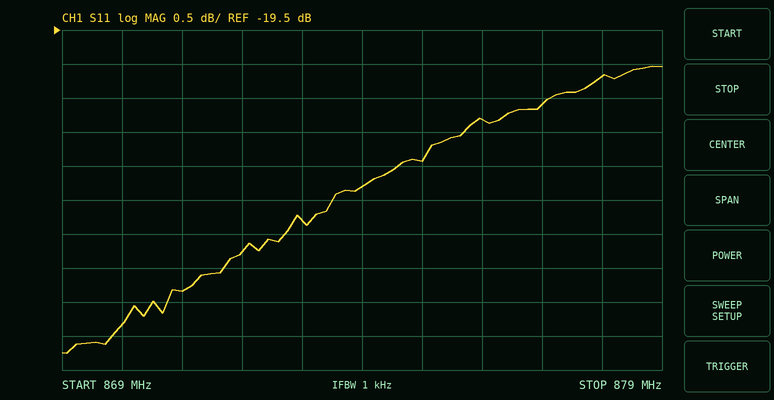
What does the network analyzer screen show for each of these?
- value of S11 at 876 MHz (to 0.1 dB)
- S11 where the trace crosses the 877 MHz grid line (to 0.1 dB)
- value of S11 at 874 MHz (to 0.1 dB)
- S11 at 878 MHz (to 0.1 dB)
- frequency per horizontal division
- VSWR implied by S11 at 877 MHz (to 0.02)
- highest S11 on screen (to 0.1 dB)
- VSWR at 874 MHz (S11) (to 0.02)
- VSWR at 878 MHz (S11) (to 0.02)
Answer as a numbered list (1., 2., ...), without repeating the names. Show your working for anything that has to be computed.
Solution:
1. -20.8 dB
2. -20.6 dB
3. -21.8 dB
4. -20.2 dB
5. 1 MHz
6. |Γ| = 10^(-20.6/20) = 0.0933; VSWR = (1 + 0.0933)/(1 − 0.0933) ≈ 1.21, so 1.20 to the nearest 0.02
7. -20.0 dB
8. |Γ| = 10^(-21.8/20) = 0.0813; VSWR = (1 + 0.0813)/(1 − 0.0813) ≈ 1.18
9. |Γ| = 10^(-20.2/20) = 0.0977; VSWR = (1 + 0.0977)/(1 − 0.0977) ≈ 1.22
